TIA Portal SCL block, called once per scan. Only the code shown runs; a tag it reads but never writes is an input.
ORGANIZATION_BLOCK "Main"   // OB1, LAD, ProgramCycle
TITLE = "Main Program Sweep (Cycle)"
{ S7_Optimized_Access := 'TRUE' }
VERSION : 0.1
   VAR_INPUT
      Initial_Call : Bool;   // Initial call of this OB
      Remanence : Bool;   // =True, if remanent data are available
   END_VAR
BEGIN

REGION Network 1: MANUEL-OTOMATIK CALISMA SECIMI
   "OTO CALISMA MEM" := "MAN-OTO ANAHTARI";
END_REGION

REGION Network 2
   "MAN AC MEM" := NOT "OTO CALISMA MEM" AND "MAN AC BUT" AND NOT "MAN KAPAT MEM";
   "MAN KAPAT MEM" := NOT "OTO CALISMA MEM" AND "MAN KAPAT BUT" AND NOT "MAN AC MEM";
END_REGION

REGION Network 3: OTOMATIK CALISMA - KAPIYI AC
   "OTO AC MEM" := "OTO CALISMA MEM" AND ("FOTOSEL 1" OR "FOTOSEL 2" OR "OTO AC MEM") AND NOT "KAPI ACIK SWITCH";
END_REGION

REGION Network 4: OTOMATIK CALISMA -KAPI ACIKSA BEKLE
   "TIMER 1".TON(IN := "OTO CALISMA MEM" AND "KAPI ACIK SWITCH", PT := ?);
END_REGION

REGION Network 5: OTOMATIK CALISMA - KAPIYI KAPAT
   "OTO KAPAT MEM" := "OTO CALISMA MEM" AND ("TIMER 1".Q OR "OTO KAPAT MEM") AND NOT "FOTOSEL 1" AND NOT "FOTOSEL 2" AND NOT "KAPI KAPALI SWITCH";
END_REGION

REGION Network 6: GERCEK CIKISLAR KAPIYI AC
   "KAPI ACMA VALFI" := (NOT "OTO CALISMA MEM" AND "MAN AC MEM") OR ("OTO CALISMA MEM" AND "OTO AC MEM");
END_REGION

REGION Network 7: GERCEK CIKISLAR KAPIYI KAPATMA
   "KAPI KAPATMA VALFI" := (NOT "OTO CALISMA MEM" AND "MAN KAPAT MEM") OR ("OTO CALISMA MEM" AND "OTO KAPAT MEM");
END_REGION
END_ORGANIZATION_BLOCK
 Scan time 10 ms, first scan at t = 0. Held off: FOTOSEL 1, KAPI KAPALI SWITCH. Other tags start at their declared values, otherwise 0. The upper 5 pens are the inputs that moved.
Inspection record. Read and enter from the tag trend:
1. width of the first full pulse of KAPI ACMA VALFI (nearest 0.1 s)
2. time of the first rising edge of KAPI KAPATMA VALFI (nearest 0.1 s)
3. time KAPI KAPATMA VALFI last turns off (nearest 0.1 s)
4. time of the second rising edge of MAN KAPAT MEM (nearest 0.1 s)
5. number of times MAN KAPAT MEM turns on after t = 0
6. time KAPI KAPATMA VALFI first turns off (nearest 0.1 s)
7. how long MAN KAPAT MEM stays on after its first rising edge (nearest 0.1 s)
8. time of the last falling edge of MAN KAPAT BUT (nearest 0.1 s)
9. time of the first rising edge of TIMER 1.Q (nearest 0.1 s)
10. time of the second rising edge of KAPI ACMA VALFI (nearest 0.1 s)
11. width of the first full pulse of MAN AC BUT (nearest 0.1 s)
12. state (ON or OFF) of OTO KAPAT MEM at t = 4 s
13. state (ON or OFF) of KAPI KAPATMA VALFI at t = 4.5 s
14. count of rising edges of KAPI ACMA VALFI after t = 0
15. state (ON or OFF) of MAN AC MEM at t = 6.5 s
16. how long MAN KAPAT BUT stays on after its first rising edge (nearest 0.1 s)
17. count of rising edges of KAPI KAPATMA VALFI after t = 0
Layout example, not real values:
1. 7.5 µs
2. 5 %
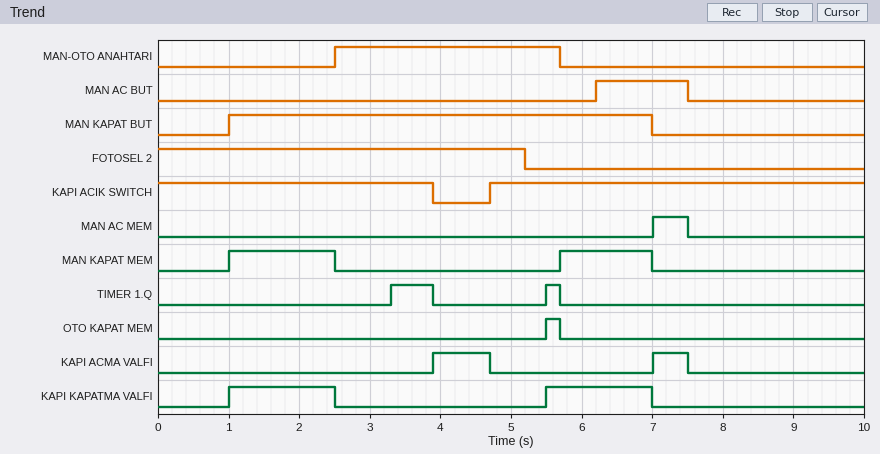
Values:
1. 0.8 s
2. 1.0 s
3. 7.0 s
4. 5.7 s
5. 2
6. 2.5 s
7. 1.5 s
8. 7.0 s
9. 3.3 s
10. 7.0 s
11. 1.3 s
12. OFF
13. OFF
14. 2
15. OFF
16. 6.0 s
17. 2
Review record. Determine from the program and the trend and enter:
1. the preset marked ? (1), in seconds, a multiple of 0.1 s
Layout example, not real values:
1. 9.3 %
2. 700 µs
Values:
1. 0.8 s
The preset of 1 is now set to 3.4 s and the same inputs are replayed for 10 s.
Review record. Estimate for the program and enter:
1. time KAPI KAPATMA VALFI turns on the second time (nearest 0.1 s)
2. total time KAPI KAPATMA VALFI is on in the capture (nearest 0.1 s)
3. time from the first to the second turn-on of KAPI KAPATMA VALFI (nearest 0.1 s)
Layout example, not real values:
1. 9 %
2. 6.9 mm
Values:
1. 5.7 s
2. 2.8 s
3. 4.7 s
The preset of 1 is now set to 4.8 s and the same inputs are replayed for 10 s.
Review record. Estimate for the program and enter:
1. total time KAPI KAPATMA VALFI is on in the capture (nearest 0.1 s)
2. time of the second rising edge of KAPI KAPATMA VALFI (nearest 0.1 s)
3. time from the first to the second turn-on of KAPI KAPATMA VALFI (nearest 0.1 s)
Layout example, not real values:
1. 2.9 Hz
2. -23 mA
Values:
1. 2.8 s
2. 5.7 s
3. 4.7 s
